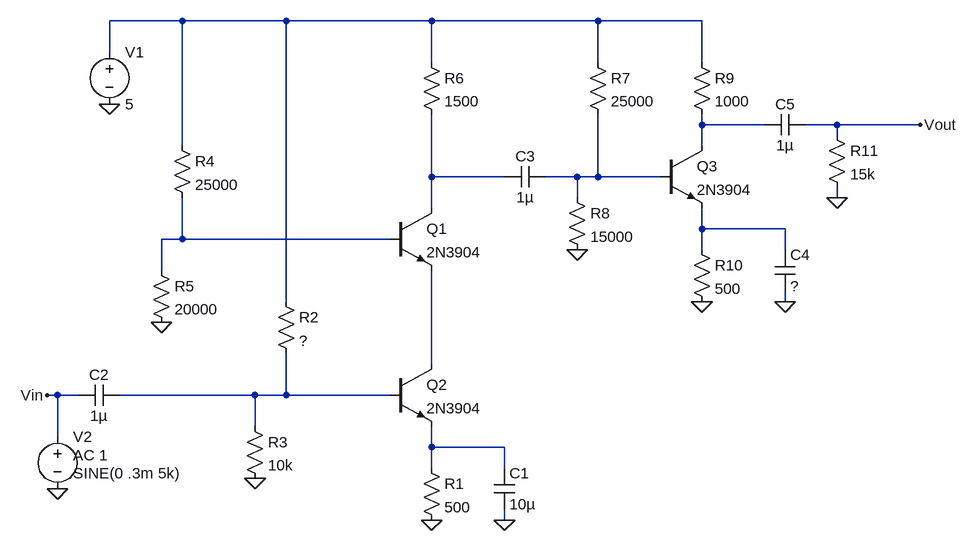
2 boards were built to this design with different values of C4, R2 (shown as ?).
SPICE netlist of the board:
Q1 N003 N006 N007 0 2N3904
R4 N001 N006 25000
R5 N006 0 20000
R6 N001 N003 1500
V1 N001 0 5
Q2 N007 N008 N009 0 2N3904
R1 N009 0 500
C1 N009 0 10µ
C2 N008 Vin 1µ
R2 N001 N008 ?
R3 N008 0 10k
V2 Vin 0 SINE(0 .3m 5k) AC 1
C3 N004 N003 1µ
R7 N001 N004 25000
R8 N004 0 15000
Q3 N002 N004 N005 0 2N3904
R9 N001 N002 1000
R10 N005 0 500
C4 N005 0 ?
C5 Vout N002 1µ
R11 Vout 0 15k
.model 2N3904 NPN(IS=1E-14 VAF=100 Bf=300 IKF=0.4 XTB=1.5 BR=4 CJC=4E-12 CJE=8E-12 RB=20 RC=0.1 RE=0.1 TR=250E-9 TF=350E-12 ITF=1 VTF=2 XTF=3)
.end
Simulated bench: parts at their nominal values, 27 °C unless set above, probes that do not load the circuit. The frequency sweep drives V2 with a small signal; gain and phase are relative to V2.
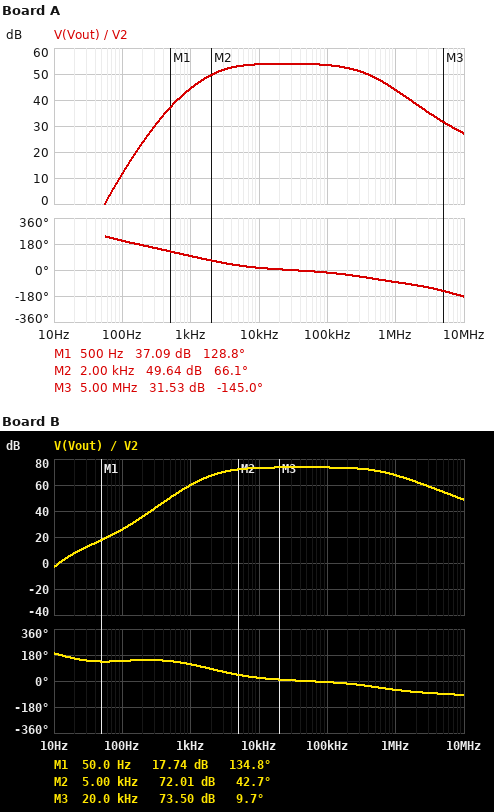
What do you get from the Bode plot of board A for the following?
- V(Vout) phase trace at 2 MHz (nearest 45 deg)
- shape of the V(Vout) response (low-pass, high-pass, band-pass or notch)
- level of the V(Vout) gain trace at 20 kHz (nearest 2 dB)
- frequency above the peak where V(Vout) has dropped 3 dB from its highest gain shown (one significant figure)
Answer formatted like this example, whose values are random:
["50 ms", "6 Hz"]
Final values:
["-90 deg", "band-pass", "54 dB", "300 kHz"]
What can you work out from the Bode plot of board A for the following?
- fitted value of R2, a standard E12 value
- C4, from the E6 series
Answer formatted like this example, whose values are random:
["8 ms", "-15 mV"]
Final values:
["12 kΩ", "33 µF"]
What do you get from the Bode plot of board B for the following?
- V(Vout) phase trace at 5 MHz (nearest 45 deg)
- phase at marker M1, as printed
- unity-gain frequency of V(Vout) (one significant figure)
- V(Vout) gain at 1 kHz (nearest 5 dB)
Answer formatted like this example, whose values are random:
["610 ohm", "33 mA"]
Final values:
["-90 deg", "134.8 deg", "10 Hz", "60 dB"]
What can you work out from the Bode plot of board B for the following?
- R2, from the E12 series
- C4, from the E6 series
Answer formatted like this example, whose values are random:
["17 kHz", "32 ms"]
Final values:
["22 kΩ", "3.3 µF"]
